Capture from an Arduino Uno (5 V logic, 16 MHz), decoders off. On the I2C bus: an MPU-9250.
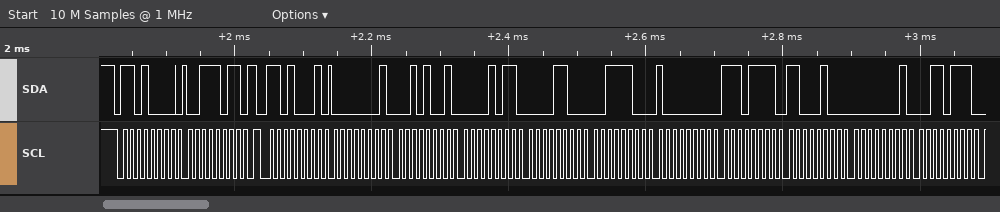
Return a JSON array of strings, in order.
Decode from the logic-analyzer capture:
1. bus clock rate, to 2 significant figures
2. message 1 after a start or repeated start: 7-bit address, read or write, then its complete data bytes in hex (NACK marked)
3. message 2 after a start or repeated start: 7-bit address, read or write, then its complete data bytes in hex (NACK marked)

["100 kHz", "0x68 write: 3B", "0x68 read: 01 29 0B 0C 3C 80 EF C4 01 37"]
